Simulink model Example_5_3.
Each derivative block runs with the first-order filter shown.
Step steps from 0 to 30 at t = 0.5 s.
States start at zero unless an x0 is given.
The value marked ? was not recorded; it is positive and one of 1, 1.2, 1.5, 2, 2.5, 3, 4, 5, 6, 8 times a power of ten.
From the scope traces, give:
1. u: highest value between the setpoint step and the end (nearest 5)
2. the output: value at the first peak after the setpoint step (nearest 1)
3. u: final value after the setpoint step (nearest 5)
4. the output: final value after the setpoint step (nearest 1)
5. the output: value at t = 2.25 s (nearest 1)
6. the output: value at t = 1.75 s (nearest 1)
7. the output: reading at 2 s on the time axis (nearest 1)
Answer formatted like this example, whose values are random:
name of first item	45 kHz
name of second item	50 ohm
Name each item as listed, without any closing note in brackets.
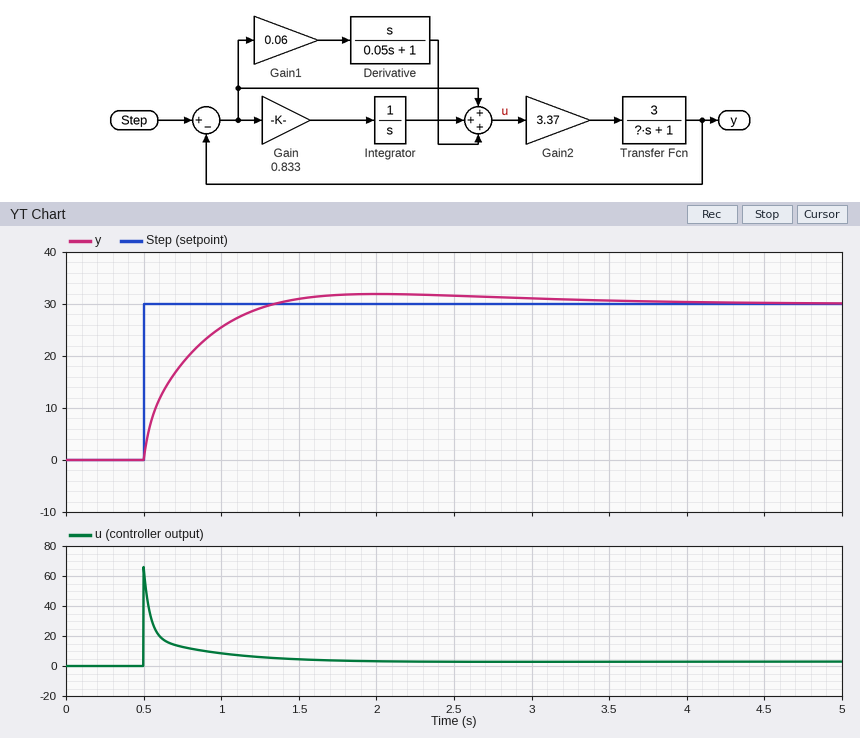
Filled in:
u: highest value between the setpoint step and the end	65
the output: value at the first peak after the setpoint step	32
u: final value after the setpoint step	5
the output: final value after the setpoint step	30
the output: value at t = 2.25 s	32
the output: value at t = 1.75 s	32
the output: reading at 2 s on the time axis	32
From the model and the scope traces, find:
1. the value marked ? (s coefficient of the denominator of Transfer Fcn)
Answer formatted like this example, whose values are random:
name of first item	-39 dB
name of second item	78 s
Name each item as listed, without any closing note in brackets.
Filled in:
the value marked ?	3
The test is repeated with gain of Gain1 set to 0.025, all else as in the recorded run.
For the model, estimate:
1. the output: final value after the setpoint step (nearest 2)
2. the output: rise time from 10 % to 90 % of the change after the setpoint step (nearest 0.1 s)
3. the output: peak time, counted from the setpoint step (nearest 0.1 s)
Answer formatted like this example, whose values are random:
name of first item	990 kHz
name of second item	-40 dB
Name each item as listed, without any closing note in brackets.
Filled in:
the output: final value after the setpoint step	30
the output: rise time from 10 % to 90 % of the change after the setpoint step	0.5 s
the output: peak time, counted from the setpoint step	1.4 s
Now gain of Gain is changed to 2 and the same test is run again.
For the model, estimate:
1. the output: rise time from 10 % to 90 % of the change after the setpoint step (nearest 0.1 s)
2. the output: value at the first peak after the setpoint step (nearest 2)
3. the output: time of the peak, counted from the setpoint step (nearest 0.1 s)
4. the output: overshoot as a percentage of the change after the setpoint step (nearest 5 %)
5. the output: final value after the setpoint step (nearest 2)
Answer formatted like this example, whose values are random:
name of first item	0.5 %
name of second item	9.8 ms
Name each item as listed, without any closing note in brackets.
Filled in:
the output: rise time from 10 % to 90 % of the change after the setpoint step	0.4 s
the output: value at the first peak after the setpoint step	34
the output: time of the peak, counted from the setpoint step	1.0 s
the output: overshoot as a percentage of the change after the setpoint step	15 %
the output: final value after the setpoint step	30
